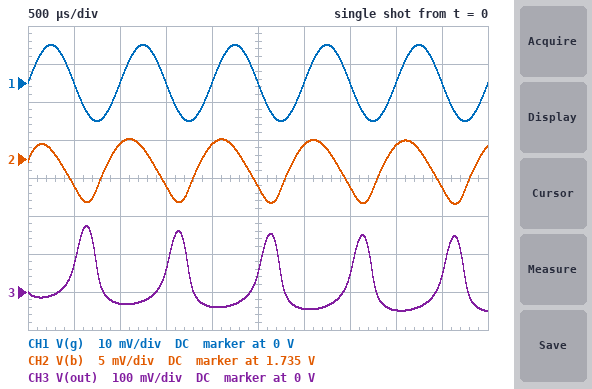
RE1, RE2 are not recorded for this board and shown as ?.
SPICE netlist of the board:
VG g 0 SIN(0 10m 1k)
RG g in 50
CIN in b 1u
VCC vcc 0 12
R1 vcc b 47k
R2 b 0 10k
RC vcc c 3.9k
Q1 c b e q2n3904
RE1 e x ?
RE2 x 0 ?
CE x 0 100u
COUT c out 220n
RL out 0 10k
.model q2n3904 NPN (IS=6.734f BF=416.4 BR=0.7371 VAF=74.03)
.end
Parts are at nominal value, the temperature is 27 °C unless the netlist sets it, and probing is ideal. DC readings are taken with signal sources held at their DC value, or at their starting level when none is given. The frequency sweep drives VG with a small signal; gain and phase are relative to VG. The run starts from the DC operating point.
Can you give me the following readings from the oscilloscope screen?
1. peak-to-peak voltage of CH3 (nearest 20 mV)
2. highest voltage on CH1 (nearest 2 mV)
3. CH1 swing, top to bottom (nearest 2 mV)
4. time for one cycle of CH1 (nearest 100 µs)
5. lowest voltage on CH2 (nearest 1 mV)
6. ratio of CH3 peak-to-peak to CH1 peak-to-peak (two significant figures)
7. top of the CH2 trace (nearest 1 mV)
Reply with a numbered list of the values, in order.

1. 220 mV
2. 10 mV
3. 20 mV
4. 1.0 ms
5. 1.729 V
6. 11
7. 1.738 V
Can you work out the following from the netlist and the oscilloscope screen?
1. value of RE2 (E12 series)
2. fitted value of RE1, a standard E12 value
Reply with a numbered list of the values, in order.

1. 330 Ω
2. 39 Ω
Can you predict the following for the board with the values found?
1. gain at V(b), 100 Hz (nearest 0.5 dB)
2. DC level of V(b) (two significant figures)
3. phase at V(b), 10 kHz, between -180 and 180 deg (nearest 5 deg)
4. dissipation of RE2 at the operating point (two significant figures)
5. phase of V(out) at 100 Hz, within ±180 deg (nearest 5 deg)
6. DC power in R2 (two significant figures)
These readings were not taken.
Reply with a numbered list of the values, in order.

1. -27.5 dB
2. 1.7 V
3. 10 deg
4. 2.6 mW
5. -55 deg
6. 300 µW
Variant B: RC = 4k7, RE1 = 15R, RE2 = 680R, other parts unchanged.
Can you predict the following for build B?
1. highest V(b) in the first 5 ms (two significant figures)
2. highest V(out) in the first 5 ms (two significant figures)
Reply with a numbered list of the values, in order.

1. 2.1 V
2. 1.1 V
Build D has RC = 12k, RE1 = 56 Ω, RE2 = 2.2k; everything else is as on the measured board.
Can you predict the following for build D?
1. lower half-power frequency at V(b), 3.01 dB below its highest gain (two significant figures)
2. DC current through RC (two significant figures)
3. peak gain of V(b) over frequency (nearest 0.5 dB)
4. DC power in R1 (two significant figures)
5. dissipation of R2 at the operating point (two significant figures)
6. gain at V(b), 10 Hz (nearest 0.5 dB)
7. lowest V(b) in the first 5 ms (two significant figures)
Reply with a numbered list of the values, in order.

1. 24 Hz
2. 640 µA
3. 0 dB
4. 2.1 mW
5. 440 µW
6. -7.5 dB
7. 2.1 V
